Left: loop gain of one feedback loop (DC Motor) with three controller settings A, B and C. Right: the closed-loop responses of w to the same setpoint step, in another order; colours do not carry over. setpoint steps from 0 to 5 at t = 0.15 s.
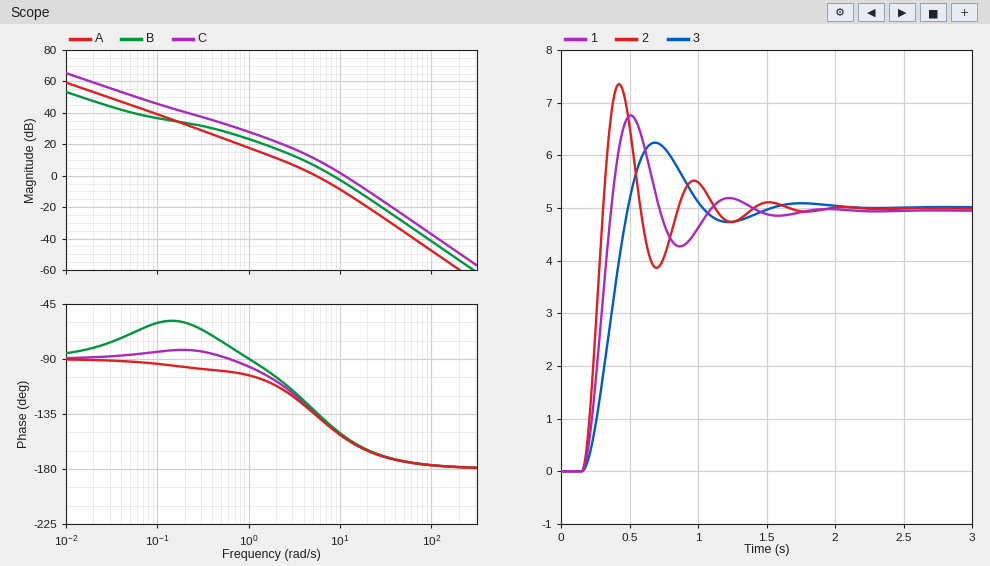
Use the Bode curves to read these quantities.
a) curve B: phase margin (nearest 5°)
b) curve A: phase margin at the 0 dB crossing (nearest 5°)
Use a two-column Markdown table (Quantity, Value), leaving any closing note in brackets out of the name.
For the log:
| Quantity | Value |
|---|---|
| curve B: phase margin | 35° |
| curve A: phase margin at the 0 dB crossing | 45° |
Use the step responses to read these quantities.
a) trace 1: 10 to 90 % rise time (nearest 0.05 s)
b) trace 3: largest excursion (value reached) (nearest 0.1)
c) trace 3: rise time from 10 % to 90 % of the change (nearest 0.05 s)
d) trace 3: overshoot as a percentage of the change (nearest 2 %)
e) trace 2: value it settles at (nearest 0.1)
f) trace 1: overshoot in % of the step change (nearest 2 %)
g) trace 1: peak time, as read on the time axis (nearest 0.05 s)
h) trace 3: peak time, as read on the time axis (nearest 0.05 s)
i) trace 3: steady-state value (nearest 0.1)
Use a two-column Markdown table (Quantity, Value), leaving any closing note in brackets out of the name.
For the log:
| Quantity | Value |
|---|---|
| trace 1: 10 to 90 % rise time | 0.15 s |
| trace 3: largest excursion (value reached) | 6.2 |
| trace 3: rise time from 10 % to 90 % of the change | 0.25 s |
| trace 3: overshoot as a percentage of the change | 24 % |
| trace 2: value it settles at | 5.0 |
| trace 1: overshoot in % of the step change | 36 % |
| trace 1: peak time, as read on the time axis | 0.50 s |
| trace 3: peak time, as read on the time axis | 0.70 s |
| trace 3: steady-state value | 5.0 |
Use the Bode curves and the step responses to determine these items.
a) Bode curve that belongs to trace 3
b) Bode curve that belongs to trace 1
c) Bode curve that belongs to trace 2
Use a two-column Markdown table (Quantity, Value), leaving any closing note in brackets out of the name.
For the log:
| Quantity | Value |
|---|---|
| Bode curve that belongs to trace 3 | A |
| Bode curve that belongs to trace 1 | B |
| Bode curve that belongs to trace 2 | C |
